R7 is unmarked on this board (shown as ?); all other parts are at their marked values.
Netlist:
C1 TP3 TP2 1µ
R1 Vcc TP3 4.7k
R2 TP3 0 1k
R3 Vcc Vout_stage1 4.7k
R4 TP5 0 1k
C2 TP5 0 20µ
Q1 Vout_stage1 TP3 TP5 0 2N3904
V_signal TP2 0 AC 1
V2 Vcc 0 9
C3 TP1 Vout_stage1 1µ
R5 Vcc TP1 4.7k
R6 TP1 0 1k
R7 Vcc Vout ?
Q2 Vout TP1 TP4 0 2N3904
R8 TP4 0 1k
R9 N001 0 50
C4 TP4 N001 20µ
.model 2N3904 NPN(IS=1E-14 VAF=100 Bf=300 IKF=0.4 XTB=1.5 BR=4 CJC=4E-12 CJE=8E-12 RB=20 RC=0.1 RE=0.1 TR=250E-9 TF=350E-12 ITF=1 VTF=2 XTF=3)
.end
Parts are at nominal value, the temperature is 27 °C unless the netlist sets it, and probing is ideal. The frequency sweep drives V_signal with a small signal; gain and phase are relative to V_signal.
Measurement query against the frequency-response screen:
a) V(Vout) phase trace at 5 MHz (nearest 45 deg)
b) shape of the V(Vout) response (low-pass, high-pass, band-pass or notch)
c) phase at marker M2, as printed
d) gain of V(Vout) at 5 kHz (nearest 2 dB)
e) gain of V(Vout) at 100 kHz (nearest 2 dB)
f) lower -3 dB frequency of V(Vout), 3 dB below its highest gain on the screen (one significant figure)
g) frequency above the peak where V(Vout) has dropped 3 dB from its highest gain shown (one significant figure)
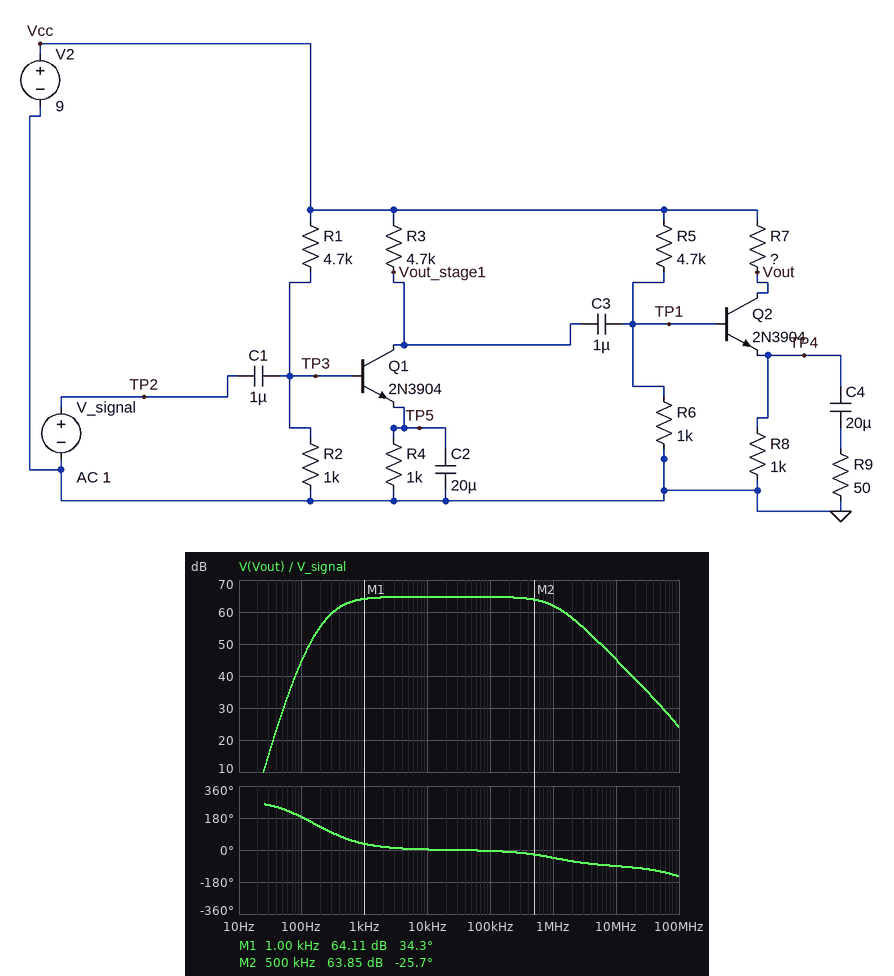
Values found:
-90 deg
band-pass
-25.7 deg
64 dB
64 dB
400 Hz
1 MHz
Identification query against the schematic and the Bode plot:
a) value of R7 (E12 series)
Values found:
5.6 kΩ
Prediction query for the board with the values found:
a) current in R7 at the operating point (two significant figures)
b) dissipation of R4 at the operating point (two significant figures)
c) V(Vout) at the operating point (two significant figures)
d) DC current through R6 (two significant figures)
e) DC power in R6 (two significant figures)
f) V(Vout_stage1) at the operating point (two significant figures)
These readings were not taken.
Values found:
920 µA
850 µW
3.8 V
1.6 mA
2.5 mW
4.7 V
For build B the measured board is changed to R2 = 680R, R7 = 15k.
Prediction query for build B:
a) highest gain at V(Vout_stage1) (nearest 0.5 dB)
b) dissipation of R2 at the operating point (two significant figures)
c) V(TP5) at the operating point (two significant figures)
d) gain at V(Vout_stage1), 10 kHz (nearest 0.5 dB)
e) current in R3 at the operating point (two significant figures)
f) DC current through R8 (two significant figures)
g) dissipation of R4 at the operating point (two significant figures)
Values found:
17.0 dB
1.9 mW
500 mV
7.5 dB
500 µA
750 µA
250 µW
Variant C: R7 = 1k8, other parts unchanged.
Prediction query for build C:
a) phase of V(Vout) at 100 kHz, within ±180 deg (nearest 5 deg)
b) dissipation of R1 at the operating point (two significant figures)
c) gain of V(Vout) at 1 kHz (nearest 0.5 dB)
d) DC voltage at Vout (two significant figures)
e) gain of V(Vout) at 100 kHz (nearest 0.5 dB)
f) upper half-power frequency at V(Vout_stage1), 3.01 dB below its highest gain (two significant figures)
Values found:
0 deg
12 mW
54.5 dB
7.3 V
55.0 dB
3.5 MHz
